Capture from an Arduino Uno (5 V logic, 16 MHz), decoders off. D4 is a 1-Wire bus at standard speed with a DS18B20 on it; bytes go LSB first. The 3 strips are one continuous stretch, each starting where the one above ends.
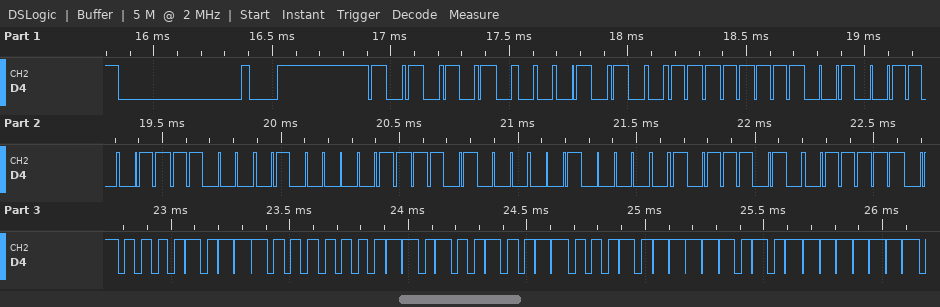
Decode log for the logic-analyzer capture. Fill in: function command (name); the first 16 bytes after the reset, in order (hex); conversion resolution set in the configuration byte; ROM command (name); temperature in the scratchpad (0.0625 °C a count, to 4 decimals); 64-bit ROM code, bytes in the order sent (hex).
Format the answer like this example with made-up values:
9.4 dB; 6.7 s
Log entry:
Read Scratchpad; 55 28 FF 64 1E 82 17 04 5D BE D0 01 4B 46 5F FF; 11 bits; Match ROM; 29.0000 °C; 28 FF 64 1E 82 17 04 5D
